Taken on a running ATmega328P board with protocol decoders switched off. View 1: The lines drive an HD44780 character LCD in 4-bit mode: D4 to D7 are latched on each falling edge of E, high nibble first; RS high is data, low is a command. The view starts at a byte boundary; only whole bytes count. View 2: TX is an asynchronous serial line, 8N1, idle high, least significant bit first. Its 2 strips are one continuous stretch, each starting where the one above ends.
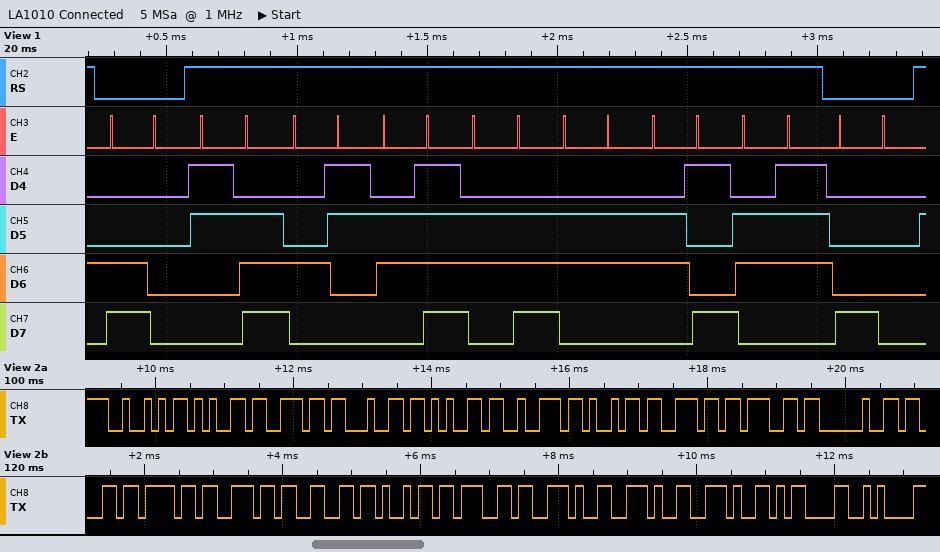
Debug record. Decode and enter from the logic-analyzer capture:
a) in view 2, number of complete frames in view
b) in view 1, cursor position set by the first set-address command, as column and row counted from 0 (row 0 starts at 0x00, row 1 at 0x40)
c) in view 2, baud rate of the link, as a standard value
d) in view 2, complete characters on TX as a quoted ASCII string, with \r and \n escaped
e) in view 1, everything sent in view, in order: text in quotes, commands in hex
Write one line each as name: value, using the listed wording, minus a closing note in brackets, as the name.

in view 2, number of complete frames in view: 21
in view 1, cursor position set by the first set-address command, as column and row counted from 0: column 0, row 1
in view 2, baud rate of the link, as a standard value: 9600 baud
in view 2, complete characters on TX as a quoted ASCII string, with \r and \n escaped: "Rendering config...\r\n"
in view 1, everything sent in view, in order: text in quotes, commands in hex: 0xC0 ">Config" 0x80
